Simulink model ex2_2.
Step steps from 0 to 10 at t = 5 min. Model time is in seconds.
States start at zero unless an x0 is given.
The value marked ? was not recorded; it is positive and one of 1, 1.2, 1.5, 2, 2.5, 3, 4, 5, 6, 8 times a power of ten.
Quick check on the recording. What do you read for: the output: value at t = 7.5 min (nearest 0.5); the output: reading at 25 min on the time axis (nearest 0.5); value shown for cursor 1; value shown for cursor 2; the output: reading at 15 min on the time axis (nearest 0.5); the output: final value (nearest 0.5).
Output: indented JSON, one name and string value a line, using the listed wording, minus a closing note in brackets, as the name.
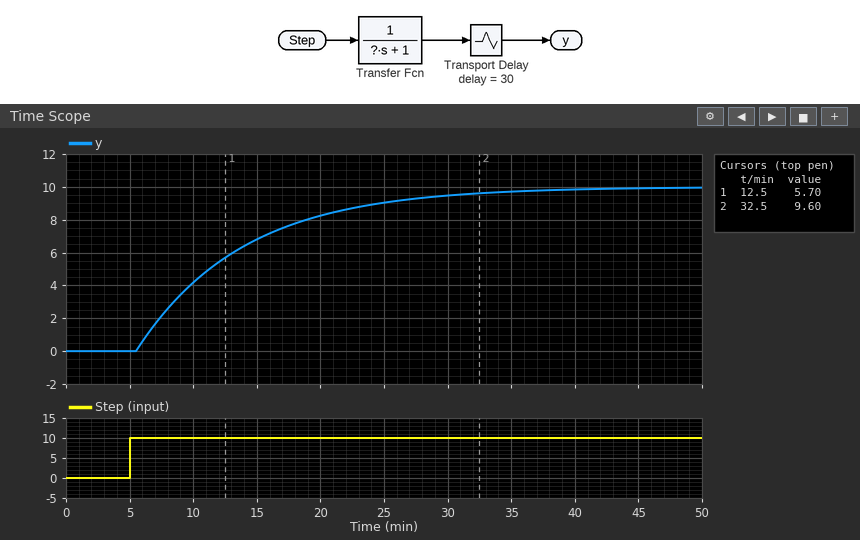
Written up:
{
  "the output: value at t = 7.5 min": "2.0",
  "the output: reading at 25 min on the time axis": "9.0",
  "value shown for cursor 1": "5.70",
  "value shown for cursor 2": "9.60",
  "the output: reading at 15 min on the time axis": "7.0",
  "the output: final value": "10.0"
}
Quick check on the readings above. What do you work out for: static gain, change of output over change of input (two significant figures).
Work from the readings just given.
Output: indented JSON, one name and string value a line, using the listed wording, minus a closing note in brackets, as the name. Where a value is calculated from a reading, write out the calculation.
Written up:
{
  "static gain, change of output over change of input": "(10 - 0) / (10 - 0) = 1.0"
}
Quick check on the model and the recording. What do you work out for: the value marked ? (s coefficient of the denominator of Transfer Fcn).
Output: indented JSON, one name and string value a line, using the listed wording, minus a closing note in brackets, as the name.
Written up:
{
  "the value marked ?": "500"
}
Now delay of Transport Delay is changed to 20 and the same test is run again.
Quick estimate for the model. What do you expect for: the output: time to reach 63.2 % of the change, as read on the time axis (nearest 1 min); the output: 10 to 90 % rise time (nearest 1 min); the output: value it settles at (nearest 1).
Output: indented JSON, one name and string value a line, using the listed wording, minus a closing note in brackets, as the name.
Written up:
{
  "the output: time to reach 63.2 % of the change, as read on the time axis": "14 min",
  "the output: 10 to 90 % rise time": "18 min",
  "the output: value it settles at": "10"
}
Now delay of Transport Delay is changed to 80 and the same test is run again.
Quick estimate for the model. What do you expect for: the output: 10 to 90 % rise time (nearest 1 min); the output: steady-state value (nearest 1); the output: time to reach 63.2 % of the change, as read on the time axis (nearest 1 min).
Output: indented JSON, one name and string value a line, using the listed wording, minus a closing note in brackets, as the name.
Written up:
{
  "the output: 10 to 90 % rise time": "18 min",
  "the output: steady-state value": "10",
  "the output: time to reach 63.2 % of the change, as read on the time axis": "15 min"
}
